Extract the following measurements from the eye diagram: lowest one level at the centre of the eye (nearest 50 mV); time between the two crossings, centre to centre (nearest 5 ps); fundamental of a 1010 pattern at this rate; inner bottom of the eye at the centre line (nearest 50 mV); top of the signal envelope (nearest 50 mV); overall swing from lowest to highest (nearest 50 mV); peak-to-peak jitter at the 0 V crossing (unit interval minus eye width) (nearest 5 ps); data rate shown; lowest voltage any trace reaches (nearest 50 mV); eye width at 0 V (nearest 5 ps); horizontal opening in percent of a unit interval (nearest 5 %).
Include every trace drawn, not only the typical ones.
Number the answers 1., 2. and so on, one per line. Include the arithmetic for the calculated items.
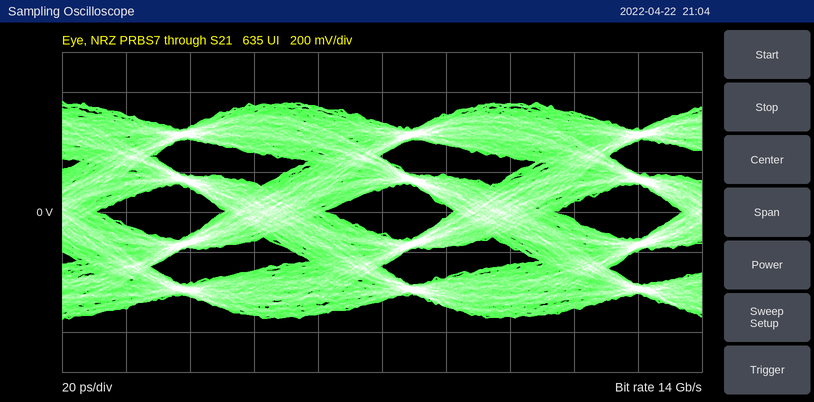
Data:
1. 100 mV
2. 70 ps
3. 7 GHz
4. -100 mV
5. 550 mV
6. 1.10 V
7. 30 ps
8. 14 Gb/s
9. -550 mV
10. 40 ps
11. 40 ps / 70 ps ≈ 57.1 %, so 55 % to the nearest 5 %
